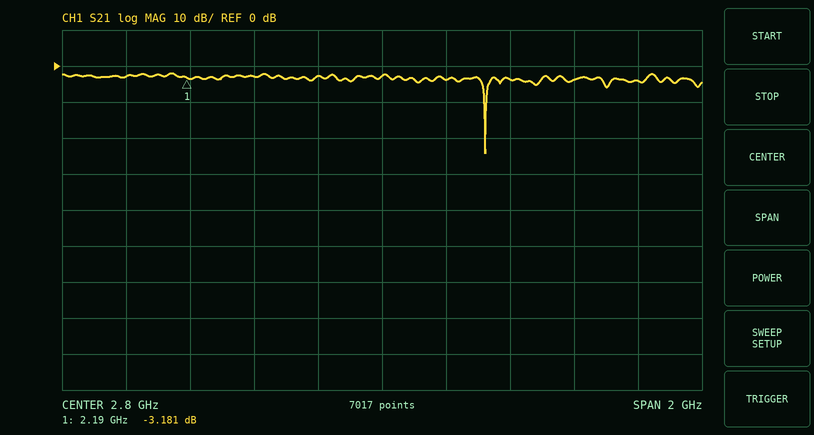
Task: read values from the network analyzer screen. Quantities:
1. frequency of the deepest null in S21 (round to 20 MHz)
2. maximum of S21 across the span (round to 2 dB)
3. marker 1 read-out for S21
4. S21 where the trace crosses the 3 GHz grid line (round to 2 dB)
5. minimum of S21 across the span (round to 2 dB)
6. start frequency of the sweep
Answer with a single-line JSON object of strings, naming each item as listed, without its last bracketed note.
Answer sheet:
{"frequency of the deepest null in S21": "3.12 GHz", "maximum of S21 across the span": "-2 dB", "marker 1 read-out for S21": "-3.181 dB", "S21 where the trace crosses the 3 GHz grid line": "-4 dB", "minimum of S21 across the span": "-24 dB", "start frequency of the sweep": "1.8 GHz"}
